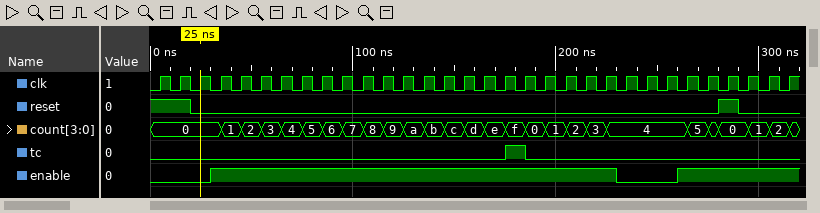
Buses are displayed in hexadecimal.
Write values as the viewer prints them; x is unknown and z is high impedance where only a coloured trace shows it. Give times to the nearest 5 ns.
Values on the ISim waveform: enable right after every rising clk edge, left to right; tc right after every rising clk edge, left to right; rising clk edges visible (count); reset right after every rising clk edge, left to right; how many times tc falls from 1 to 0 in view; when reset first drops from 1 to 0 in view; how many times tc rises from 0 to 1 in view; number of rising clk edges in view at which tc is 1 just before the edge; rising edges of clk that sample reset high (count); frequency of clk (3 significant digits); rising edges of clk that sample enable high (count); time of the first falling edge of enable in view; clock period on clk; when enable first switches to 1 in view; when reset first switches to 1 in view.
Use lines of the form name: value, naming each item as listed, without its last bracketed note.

enable right after every rising clk edge, left to right: 0 0 0 1 1 1 1 1 1 1 1 1 1 1 1 1 1 1 1 1 1 1 1 0 0 0 1 1 1 1 1 1
tc right after every rising clk edge, left to right: 0 0 0 0 0 0 0 0 0 0 0 0 0 0 0 0 0 1 0 0 0 0 0 0 0 0 0 0 0 0 0 0
rising clk edges visible: 32
reset right after every rising clk edge, left to right: 1 1 0 0 0 0 0 0 0 0 0 0 0 0 0 0 0 0 0 0 0 0 0 0 0 0 0 0 1 0 0 0
how many times tc falls from 1 to 0 in view: 1
when reset first drops from 1 to 0 in view: 20 ns
how many times tc rises from 0 to 1 in view: 1
number of rising clk edges in view at which tc is 1 just before the edge: 1
rising edges of clk that sample reset high: 3
frequency of clk: 100 MHz
rising edges of clk that sample enable high: 26
time of the first falling edge of enable in view: 230 ns
clock period on clk: 10 ns
when enable first switches to 1 in view: 30 ns
when reset first switches to 1 in view: 280 ns
